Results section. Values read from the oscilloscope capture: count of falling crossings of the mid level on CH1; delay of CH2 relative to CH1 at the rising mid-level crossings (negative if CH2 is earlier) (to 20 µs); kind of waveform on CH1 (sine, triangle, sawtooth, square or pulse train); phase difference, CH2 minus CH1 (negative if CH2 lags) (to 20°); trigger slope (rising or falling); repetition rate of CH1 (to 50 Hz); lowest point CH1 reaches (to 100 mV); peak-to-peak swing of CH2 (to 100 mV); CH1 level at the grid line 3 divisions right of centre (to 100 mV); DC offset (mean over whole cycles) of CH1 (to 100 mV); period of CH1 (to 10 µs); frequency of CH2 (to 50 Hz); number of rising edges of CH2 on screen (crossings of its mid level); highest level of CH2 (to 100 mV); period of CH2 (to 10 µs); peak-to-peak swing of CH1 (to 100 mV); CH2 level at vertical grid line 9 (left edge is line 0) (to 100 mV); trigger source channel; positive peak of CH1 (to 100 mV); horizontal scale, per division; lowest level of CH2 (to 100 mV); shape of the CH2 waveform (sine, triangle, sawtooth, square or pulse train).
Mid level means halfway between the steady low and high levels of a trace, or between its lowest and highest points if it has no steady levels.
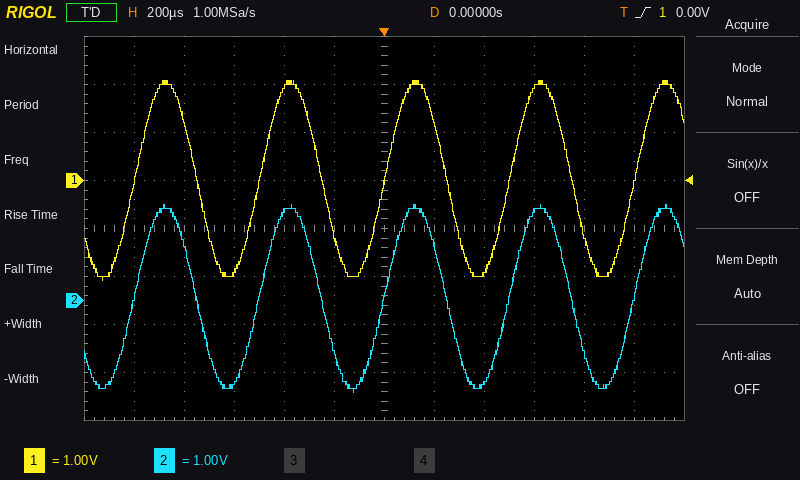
4
0 µs
sine
0°
rising
2.00 kHz
-2.1 V
3.9 V
1.9 V
0.0 V
500 µs
2.00 kHz
5
2.0 V
500 µs
4.2 V
1.8 V
CH1
2.1 V
200 µs
-1.9 V
sine
